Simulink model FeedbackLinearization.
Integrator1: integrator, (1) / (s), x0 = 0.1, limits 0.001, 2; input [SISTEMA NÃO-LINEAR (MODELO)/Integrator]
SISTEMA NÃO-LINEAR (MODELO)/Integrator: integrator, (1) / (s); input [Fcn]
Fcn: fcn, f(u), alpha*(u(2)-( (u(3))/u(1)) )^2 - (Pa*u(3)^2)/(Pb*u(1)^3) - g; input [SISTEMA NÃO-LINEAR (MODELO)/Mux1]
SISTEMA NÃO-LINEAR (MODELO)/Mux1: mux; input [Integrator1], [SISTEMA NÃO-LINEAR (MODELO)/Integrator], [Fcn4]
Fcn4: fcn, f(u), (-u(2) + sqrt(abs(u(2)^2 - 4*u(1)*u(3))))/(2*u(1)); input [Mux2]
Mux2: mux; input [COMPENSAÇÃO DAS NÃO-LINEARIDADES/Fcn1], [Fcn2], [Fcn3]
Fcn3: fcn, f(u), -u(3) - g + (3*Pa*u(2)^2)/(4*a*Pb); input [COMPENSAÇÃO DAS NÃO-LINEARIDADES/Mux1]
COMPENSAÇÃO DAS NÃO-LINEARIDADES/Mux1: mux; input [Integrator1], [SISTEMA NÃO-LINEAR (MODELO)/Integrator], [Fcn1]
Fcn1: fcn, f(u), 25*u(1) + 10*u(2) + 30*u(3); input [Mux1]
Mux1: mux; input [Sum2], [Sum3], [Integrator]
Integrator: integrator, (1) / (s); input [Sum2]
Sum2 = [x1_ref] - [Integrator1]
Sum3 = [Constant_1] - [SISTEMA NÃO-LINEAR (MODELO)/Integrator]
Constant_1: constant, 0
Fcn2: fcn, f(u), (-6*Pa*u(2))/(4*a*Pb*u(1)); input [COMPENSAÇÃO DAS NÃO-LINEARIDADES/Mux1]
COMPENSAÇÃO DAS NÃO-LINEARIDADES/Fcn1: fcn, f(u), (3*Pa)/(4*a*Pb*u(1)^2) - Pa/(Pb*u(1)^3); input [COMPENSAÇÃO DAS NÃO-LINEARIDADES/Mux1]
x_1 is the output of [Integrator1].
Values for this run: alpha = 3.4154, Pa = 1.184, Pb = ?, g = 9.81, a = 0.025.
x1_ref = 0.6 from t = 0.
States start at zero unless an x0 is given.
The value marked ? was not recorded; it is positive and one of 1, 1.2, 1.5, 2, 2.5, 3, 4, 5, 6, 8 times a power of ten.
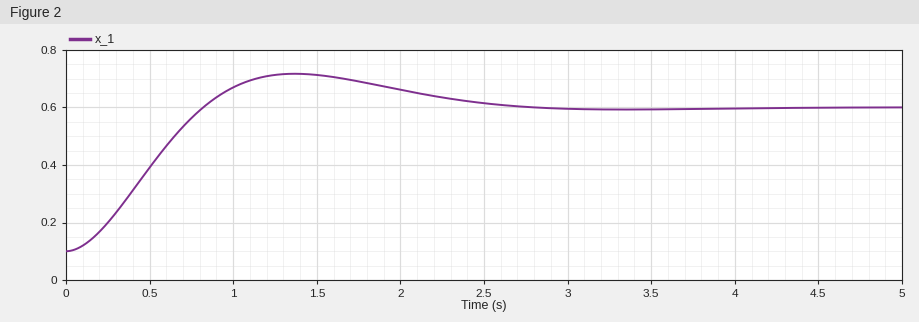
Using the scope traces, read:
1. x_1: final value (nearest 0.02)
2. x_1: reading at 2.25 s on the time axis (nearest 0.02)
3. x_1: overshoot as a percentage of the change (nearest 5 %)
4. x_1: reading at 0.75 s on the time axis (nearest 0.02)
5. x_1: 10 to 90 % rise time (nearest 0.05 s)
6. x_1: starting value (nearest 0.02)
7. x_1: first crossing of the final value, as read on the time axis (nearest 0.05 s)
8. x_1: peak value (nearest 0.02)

0.60
0.64
25 %
0.56
0.55 s
0.10
0.80 s
0.72
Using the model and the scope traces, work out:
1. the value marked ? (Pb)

8
